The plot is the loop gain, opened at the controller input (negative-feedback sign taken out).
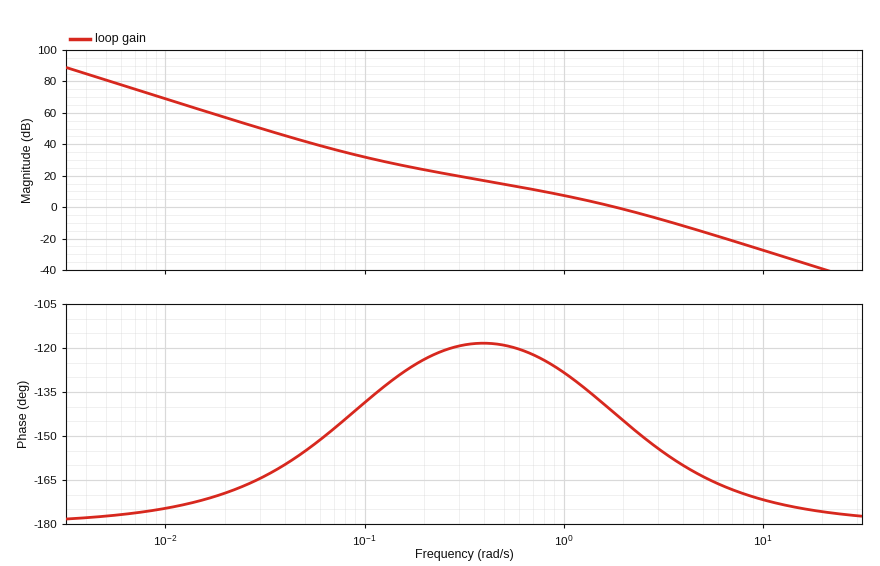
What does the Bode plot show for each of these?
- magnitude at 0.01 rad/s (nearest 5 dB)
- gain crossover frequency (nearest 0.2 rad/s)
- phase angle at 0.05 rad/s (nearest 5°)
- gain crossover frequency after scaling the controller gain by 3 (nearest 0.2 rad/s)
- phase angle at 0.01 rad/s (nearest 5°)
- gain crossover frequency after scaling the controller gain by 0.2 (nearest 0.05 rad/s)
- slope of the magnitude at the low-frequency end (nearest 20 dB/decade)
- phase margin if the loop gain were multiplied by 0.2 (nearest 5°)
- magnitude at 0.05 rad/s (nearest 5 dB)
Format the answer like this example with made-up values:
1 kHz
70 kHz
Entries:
70 dB
1.8 rad/s
-155°
3.4 rad/s
-175°
0.55 rad/s
-40 dB/decade
60°
40 dB
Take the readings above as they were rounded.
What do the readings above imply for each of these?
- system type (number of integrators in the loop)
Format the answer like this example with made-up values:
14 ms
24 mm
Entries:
2
